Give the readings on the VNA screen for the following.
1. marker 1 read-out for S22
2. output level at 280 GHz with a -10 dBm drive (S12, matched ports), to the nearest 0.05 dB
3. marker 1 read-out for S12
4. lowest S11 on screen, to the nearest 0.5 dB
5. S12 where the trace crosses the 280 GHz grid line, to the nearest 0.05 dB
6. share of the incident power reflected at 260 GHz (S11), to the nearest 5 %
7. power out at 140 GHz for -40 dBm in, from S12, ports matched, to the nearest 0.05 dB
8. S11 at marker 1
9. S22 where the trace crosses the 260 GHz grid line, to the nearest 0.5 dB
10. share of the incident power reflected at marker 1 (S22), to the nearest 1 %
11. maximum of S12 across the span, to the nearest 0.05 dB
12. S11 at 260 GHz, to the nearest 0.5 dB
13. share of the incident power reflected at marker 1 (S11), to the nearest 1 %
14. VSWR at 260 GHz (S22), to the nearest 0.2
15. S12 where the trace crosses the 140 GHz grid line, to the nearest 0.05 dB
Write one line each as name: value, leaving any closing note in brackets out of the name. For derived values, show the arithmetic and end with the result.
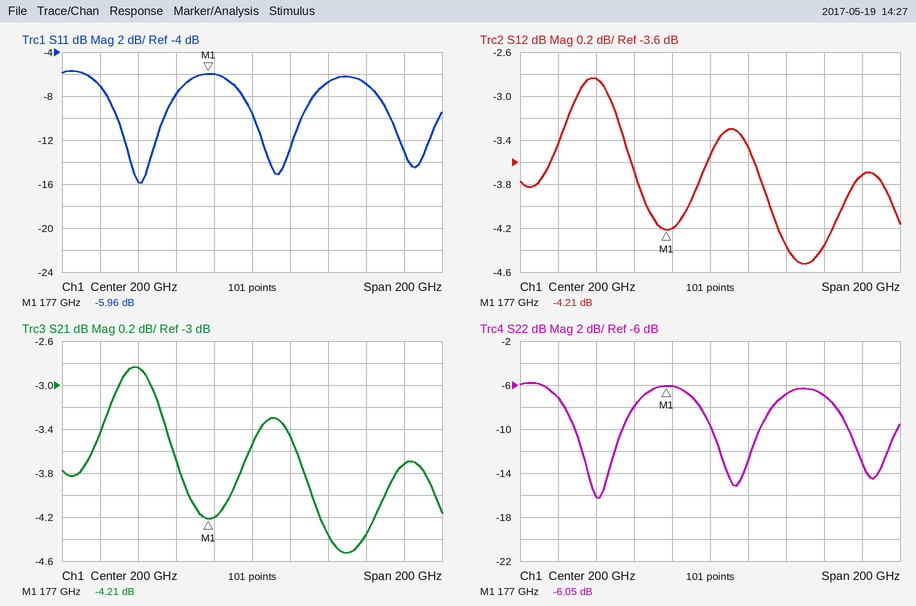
marker 1 read-out for S22: -6.05 dB
output level at 280 GHz with a -10 dBm drive (S12, matched ports), to the nearest 0.05 dB: -10 dBm + (-3.70 dB) = -13.70 dBm
marker 1 read-out for S12: -4.21 dB
lowest S11 on screen, to the nearest 0.5 dB: -16.0 dB
S12 where the trace crosses the 280 GHz grid line, to the nearest 0.05 dB: -3.70 dB
share of the incident power reflected at 260 GHz (S11), to the nearest 5 %: 10^(-7/10) ≈ 20 %
power out at 140 GHz for -40 dBm in, from S12, ports matched, to the nearest 0.05 dB: -40 dBm + (-2.85 dB) = -42.85 dBm
S11 at marker 1: -5.96 dB
S22 where the trace crosses the 260 GHz grid line, to the nearest 0.5 dB: -7.0 dB
share of the incident power reflected at marker 1 (S22), to the nearest 1 %: 10^(-6.05/10) ≈ 25 %
maximum of S12 across the span, to the nearest 0.05 dB: -2.85 dB
S11 at 260 GHz, to the nearest 0.5 dB: -7.0 dB
share of the incident power reflected at marker 1 (S11), to the nearest 1 %: 10^(-5.96/10) ≈ 25 %
VSWR at 260 GHz (S22), to the nearest 0.2: |Γ| = 10^(-7/20) = 0.4467; VSWR = (1 + 0.4467)/(1 − 0.4467) ≈ 2.6
S12 where the trace crosses the 140 GHz grid line, to the nearest 0.05 dB: -2.85 dB
